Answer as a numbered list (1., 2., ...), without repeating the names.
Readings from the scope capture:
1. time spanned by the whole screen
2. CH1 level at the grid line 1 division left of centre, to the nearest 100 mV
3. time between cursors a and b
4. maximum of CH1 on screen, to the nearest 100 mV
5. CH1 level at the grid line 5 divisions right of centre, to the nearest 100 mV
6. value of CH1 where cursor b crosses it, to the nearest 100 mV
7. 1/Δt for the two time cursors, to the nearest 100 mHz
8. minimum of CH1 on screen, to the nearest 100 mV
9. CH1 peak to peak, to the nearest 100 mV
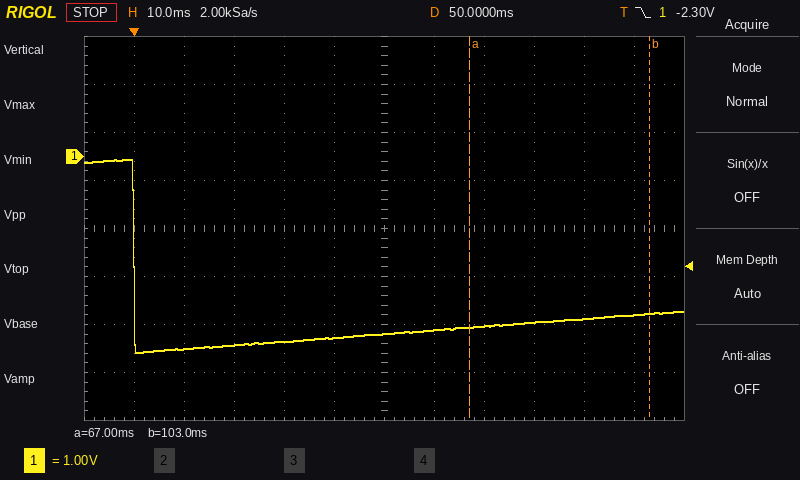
1. 120 ms
2. -3.8 V
3. 36 ms
4. -100 mV
5. -3.3 V
6. -3.3 V
7. 27.8 Hz
8. -4.1 V
9. 4.0 V
